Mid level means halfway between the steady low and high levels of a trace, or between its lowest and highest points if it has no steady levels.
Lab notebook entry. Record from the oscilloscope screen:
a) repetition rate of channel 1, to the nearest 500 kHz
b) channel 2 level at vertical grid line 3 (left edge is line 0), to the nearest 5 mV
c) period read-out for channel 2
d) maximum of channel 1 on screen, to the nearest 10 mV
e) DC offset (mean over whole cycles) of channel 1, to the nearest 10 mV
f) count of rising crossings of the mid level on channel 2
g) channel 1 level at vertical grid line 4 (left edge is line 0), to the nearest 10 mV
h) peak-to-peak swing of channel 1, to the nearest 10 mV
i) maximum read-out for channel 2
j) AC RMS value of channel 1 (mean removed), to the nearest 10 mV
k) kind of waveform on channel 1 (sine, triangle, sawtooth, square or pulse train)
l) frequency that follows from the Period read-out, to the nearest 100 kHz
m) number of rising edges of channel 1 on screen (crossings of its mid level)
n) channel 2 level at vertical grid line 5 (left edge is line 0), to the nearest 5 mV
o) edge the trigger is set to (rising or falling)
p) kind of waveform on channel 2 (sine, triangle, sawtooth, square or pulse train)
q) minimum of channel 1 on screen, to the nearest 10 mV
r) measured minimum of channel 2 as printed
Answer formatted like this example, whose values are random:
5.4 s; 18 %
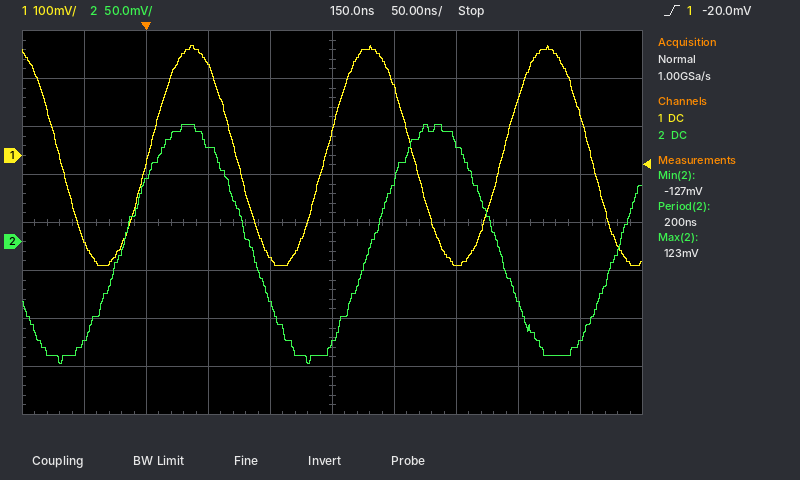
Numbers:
7.0 MHz; 100 mV; 200 ns; 230 mV; 0 mV; 3; -210 mV; 460 mV; 123 mV; 160 mV; sine; 5.0 MHz; 3; -105 mV; rising; sine; -230 mV; -127 mV
